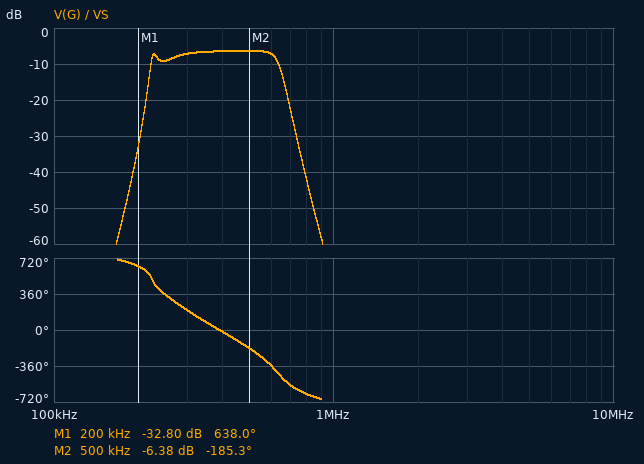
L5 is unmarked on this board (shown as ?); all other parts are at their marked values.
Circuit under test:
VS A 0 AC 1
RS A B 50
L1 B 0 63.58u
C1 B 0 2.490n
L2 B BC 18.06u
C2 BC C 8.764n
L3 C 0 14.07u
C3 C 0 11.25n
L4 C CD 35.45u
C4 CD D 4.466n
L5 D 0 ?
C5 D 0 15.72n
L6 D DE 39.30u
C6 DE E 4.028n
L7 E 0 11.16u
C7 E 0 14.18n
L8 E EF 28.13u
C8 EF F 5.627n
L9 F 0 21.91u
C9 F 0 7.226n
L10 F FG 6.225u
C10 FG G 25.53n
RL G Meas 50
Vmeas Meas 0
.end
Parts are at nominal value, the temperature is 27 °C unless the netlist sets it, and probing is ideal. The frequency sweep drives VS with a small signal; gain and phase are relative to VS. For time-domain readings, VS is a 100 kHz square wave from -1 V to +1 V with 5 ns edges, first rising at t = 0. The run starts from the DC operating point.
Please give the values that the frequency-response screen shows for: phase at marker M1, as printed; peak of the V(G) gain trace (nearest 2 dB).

638.0 deg
-6 dB
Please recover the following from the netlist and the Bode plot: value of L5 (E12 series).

15 µH
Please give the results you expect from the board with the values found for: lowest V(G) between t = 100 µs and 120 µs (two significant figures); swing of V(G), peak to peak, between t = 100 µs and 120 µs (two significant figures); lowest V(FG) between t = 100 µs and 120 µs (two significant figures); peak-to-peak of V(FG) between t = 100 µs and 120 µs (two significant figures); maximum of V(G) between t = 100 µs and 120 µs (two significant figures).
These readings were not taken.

-310 mV
630 mV
-310 mV
630 mV
310 mV
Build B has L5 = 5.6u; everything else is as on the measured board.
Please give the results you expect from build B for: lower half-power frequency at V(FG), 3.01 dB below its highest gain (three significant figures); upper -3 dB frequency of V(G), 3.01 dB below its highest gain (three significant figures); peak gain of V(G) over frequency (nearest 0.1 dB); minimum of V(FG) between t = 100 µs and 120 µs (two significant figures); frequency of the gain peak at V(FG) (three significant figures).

300 kHz
702 kHz
-6.9 dB
-300 mV
683 kHz
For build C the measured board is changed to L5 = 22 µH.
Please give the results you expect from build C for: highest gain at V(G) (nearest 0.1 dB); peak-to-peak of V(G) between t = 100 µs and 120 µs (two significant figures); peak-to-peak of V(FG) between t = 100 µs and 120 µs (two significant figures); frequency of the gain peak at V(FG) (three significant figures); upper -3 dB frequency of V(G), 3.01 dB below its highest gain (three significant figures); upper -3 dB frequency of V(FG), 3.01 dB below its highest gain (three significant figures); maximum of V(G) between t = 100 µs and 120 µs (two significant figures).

-6.9 dB
540 mV
560 mV
459 kHz
620 kHz
619 kHz
270 mV
